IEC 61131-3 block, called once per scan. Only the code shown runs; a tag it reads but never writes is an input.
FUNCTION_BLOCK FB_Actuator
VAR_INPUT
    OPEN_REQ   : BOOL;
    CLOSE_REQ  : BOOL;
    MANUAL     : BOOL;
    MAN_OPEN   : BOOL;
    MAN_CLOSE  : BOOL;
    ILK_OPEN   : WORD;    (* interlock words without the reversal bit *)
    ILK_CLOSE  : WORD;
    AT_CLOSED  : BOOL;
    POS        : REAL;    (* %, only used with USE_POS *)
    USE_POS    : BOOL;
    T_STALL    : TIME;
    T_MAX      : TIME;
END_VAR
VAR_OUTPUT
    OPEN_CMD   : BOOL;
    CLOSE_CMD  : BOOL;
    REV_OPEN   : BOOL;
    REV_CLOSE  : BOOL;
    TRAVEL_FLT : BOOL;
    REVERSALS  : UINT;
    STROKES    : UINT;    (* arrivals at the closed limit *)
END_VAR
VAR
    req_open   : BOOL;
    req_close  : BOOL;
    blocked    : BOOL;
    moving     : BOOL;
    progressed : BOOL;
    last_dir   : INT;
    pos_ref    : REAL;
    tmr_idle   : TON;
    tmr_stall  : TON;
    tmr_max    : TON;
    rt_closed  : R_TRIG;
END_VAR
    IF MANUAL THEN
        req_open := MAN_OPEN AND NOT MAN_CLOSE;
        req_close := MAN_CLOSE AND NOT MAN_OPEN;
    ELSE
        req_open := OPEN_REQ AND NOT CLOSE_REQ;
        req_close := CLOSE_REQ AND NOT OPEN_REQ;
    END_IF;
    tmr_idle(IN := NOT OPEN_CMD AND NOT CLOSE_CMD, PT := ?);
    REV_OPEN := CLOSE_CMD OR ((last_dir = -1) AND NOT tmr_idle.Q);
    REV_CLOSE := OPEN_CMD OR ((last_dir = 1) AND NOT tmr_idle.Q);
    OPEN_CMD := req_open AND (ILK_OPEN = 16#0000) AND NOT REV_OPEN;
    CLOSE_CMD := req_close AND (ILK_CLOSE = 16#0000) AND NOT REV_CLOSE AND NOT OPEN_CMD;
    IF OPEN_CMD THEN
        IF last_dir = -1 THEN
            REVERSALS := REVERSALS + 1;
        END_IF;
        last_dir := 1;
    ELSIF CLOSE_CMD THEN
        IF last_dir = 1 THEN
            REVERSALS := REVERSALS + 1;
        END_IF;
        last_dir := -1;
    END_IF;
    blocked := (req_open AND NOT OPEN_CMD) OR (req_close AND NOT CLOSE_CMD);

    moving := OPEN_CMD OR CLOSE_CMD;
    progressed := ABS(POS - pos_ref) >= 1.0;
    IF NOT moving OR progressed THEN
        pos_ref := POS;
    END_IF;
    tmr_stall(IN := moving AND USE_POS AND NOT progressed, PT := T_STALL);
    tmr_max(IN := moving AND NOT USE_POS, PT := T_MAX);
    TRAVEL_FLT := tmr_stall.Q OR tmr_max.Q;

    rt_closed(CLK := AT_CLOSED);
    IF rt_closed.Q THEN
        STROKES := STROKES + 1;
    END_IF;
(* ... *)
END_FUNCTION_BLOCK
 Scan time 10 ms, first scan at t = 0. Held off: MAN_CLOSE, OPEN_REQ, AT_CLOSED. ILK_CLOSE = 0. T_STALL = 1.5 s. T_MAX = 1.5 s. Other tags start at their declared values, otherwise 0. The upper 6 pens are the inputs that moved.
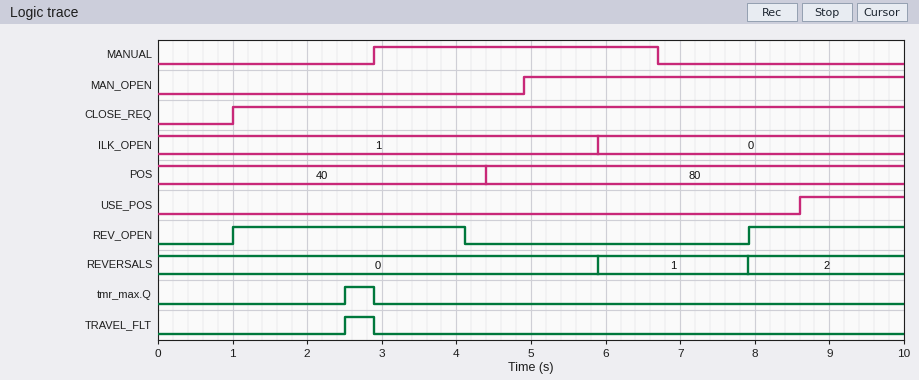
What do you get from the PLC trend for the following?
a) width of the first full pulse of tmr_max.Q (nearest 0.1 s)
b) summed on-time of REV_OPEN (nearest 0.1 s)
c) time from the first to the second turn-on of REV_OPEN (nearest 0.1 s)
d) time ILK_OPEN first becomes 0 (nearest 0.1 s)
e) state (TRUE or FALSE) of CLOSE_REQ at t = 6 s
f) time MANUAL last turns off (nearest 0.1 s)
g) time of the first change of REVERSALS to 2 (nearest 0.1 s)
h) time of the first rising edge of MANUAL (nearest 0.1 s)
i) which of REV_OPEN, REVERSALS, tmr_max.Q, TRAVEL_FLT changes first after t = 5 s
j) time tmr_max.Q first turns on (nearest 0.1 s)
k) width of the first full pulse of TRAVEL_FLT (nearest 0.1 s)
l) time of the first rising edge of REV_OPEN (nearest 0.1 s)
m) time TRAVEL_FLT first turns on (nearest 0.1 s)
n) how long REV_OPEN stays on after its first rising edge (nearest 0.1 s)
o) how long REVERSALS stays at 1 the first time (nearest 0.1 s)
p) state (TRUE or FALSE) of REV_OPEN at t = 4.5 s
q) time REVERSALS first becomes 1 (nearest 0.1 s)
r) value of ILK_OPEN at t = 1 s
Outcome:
0.4 s
5.2 s
6.9 s
5.9 s
TRUE
6.7 s
7.9 s
2.9 s
REVERSALS
2.5 s
0.4 s
1.0 s
2.5 s
3.1 s
2.0 s
FALSE
5.9 s
1
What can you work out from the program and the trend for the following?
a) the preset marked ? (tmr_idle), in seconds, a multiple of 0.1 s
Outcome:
1.2 s
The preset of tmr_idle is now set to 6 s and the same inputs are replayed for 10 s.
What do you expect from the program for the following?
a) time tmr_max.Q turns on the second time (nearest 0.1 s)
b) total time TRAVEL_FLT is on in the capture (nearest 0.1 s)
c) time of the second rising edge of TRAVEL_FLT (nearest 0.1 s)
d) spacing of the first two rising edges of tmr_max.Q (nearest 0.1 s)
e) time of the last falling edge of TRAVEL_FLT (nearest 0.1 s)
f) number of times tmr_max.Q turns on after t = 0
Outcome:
8.2 s
0.8 s
8.2 s
5.7 s
8.6 s
2
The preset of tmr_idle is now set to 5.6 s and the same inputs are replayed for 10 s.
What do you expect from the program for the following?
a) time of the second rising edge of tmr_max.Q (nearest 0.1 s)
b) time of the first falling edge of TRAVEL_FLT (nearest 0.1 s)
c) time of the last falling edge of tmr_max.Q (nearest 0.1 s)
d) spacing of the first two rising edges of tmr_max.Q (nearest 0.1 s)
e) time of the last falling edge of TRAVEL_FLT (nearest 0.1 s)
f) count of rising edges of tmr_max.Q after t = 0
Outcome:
8.2 s
2.9 s
8.6 s
5.7 s
8.6 s
2
